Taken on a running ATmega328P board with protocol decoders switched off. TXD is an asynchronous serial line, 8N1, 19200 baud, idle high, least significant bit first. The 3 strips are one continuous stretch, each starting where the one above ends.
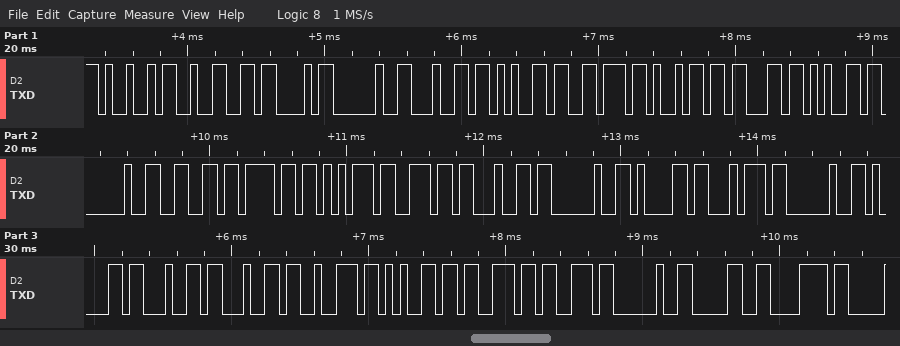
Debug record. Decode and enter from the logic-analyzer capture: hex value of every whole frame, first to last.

49 32 43 20 64 65 76 69 63 65 20 66 6F 75 6E 64 20 61 74 20 61 64 64 72 65 73 73 20 30 78
